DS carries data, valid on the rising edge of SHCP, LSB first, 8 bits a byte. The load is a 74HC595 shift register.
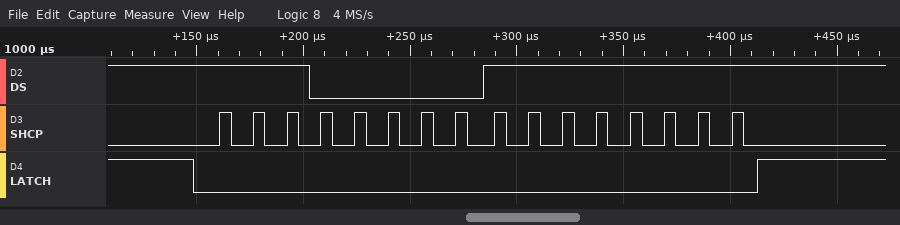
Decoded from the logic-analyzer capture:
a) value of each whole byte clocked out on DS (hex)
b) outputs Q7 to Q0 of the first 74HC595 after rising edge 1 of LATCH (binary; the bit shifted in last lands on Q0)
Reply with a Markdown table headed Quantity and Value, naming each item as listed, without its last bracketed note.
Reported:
| Quantity | Value |
|---|---|
| value of each whole byte clocked out on DS | 0x07 0xFF |
| outputs Q7 to Q0 of the first 74HC595 after rising edge 1 of LATCH | 11111111 |
